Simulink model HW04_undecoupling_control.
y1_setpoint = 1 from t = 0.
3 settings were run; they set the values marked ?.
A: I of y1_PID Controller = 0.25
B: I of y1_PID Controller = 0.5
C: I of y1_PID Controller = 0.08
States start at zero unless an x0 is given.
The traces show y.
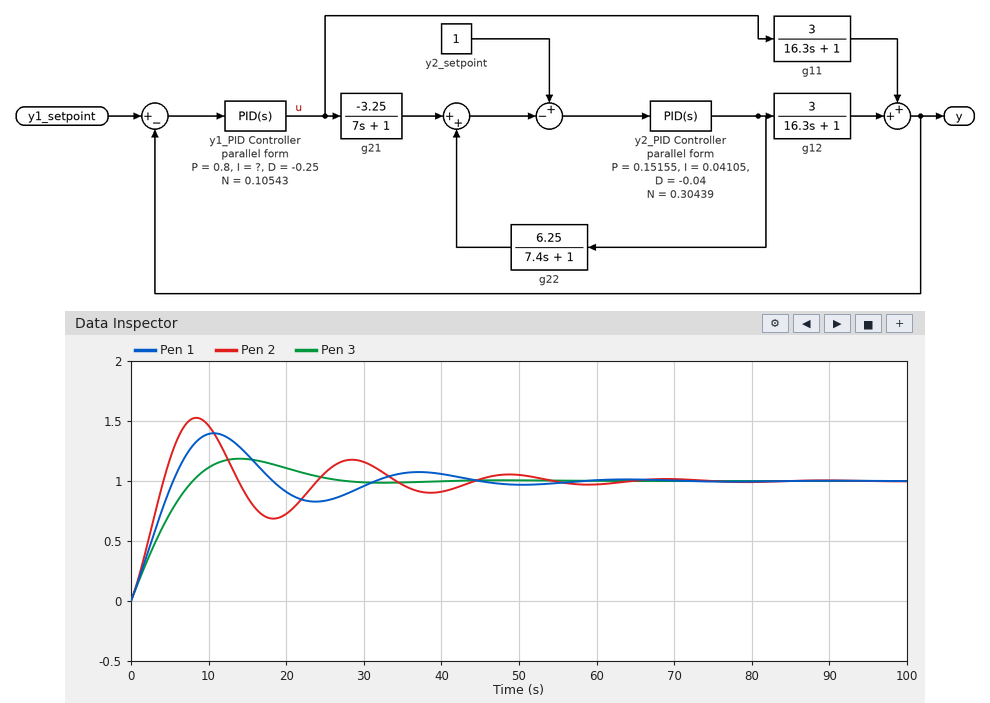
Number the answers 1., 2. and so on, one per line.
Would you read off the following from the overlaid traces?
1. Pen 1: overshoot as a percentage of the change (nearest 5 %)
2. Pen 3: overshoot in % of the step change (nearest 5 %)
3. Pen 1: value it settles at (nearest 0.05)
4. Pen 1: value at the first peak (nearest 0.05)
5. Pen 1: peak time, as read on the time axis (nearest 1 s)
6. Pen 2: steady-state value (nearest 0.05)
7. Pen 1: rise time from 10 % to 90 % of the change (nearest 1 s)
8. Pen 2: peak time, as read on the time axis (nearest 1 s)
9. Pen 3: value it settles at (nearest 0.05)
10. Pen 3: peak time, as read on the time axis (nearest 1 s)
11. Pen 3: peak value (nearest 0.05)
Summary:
1. 40 %
2. 20 %
3. 1.00
4. 1.40
5. 11 s
6. 1.00
7. 4 s
8. 8 s
9. 1.00
10. 14 s
11. 1.20
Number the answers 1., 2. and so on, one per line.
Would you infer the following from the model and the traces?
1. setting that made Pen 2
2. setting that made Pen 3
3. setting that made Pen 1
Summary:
1. B
2. C
3. A
